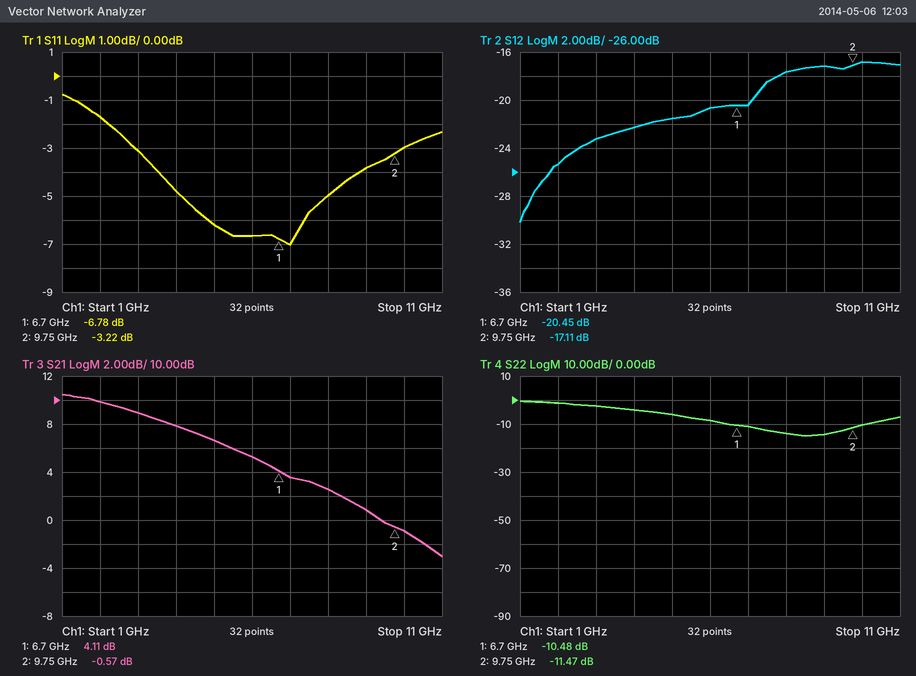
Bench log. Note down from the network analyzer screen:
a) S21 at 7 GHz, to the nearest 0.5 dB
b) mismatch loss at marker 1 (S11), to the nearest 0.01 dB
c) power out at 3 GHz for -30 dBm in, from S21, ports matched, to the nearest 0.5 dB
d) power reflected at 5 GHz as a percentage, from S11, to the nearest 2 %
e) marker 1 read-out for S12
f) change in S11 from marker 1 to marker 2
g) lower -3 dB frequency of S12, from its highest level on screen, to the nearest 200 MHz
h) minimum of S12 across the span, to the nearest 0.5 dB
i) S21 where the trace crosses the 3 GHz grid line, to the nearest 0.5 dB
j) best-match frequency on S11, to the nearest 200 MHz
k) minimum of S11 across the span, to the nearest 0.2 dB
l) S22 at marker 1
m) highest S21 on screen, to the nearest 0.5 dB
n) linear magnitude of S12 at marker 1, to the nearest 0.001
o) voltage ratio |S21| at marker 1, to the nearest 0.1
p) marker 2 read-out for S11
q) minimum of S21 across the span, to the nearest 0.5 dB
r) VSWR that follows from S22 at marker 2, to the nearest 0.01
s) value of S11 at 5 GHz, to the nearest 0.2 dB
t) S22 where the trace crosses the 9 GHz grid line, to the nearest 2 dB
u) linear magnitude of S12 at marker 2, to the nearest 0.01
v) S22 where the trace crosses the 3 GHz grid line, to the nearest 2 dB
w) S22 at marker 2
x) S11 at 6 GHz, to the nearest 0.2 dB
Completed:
3.5 dB
1.02 dB
-21.0 dBm
24 %
-20.45 dB
3.56 dB
7.2 GHz
-30.0 dB
9.0 dB
7.0 GHz
-7.0 dB
-10.48 dB
10.5 dB
0.095
1.6
-3.22 dB
-3.0 dB
1.73
-6.2 dB
-14 dB
0.14
-2 dB
-11.47 dB
-6.6 dB
